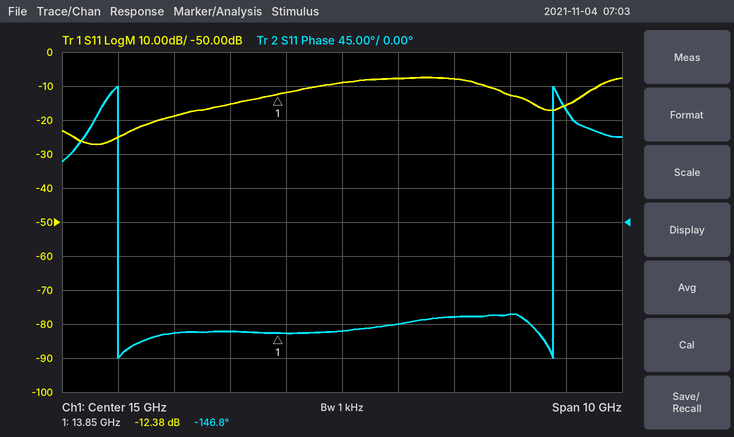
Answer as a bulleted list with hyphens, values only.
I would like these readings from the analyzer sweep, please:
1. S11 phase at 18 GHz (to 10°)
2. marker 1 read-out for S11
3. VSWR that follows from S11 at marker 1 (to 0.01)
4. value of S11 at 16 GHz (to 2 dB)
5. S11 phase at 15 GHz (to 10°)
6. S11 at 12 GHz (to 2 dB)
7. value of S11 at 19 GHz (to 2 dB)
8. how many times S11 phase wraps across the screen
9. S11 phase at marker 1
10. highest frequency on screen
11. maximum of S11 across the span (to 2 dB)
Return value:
- -120°
- -12.38 dB
- 1.63
- -8 dB
- -140°
- -18 dB
- -16 dB
- 2
- -146.8°
- 20 GHz
- -8 dB
